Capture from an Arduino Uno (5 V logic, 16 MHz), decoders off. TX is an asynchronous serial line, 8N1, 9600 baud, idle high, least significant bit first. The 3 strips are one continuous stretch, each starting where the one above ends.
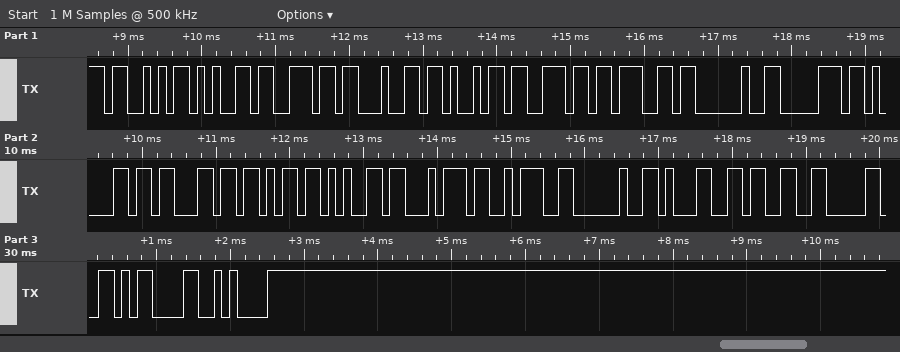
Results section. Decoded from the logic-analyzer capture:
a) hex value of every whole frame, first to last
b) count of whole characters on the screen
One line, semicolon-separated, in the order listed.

53 65 6E 64 69 6E 67 20 70 61 63 6B 65 74 3A 20 31 33 30 0D 0A; 21
